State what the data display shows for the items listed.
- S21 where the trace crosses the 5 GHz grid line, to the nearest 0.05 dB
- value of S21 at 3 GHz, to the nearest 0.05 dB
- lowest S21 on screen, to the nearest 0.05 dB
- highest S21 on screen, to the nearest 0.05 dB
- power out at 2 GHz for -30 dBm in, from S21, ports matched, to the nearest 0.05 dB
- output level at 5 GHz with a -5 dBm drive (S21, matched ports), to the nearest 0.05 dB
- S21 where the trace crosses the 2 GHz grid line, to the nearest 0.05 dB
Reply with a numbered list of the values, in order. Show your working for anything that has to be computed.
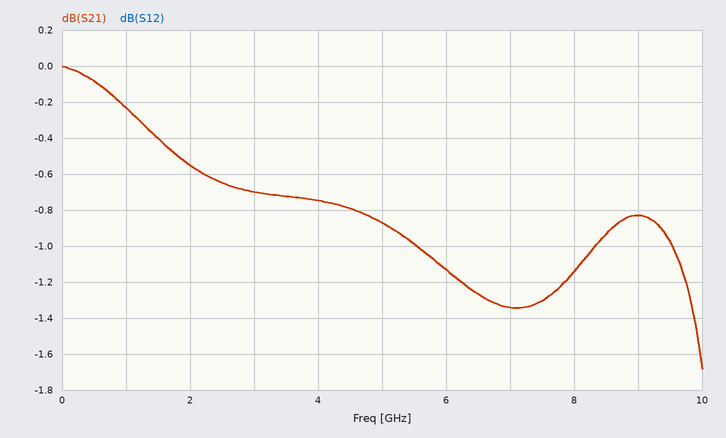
1. -0.85 dB
2. -0.70 dB
3. -1.70 dB
4. 0.00 dB
5. -30 dBm + (-0.55 dB) = -30.55 dBm
6. -5 dBm + (-0.85 dB) = -5.85 dBm
7. -0.55 dB
